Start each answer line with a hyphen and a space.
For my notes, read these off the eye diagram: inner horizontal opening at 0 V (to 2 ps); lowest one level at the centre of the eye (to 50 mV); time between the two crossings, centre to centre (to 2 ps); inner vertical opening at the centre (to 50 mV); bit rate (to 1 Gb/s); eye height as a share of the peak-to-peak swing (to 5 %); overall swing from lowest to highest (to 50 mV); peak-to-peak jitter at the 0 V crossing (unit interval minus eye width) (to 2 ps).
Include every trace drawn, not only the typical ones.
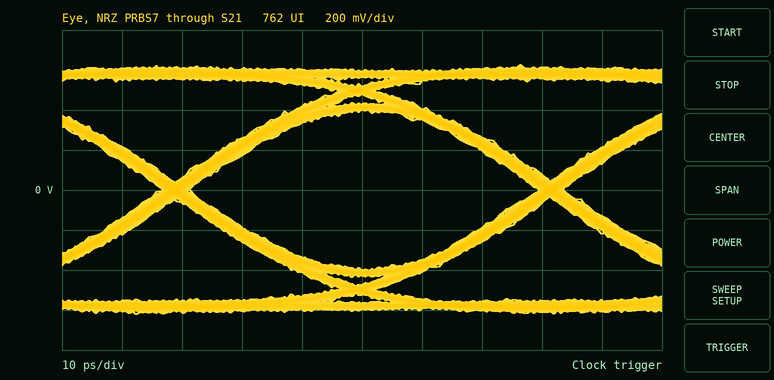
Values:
- 58 ps
- 400 mV
- 62 ps
- 800 mV
- 16 Gb/s
- 65 %
- 1.25 V
- 4 ps
